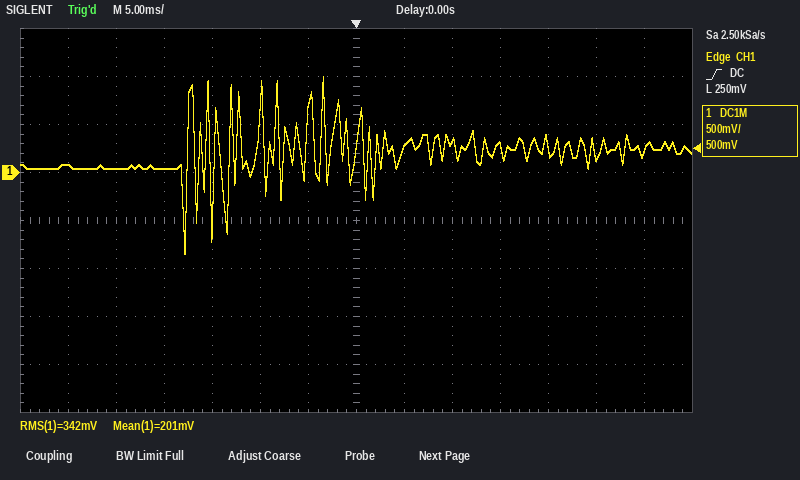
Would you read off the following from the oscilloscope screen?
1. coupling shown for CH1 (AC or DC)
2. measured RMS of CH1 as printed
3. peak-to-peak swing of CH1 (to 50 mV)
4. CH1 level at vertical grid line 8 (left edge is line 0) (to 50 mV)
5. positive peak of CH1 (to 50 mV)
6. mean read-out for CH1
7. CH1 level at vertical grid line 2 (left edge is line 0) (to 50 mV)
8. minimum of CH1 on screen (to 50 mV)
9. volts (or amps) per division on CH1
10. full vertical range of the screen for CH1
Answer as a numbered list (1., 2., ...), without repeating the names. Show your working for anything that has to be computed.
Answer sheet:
1. DC
2. 342 mV
3. 1.00 V − (-850 mV) = 1.85 V
4. 250 mV
5. 1.00 V
6. 201 mV
7. 50 mV
8. -850 mV
9. 500 mV
10. 4 V
